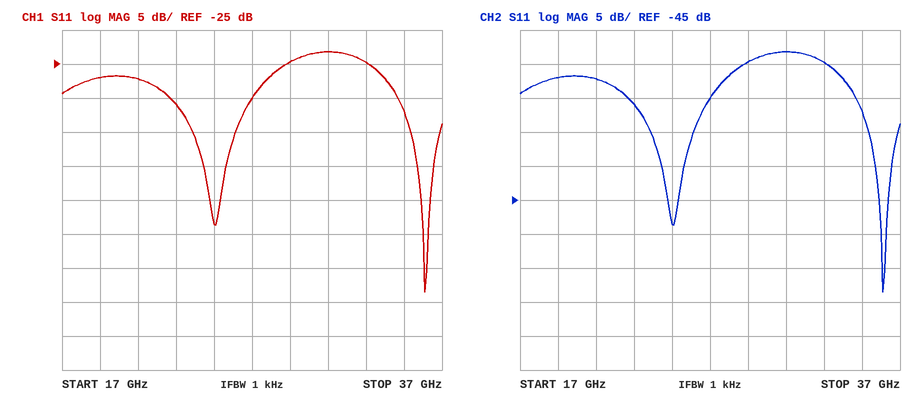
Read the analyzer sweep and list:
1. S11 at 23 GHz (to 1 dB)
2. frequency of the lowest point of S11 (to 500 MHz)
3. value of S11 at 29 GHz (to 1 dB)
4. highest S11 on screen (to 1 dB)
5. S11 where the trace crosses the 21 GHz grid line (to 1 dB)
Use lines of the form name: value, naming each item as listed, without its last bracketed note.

S11 at 23 GHz: -31 dB
frequency of the lowest point of S11: 36.0 GHz
value of S11 at 29 GHz: -25 dB
highest S11 on screen: -23 dB
S11 where the trace crosses the 21 GHz grid line: -27 dB
